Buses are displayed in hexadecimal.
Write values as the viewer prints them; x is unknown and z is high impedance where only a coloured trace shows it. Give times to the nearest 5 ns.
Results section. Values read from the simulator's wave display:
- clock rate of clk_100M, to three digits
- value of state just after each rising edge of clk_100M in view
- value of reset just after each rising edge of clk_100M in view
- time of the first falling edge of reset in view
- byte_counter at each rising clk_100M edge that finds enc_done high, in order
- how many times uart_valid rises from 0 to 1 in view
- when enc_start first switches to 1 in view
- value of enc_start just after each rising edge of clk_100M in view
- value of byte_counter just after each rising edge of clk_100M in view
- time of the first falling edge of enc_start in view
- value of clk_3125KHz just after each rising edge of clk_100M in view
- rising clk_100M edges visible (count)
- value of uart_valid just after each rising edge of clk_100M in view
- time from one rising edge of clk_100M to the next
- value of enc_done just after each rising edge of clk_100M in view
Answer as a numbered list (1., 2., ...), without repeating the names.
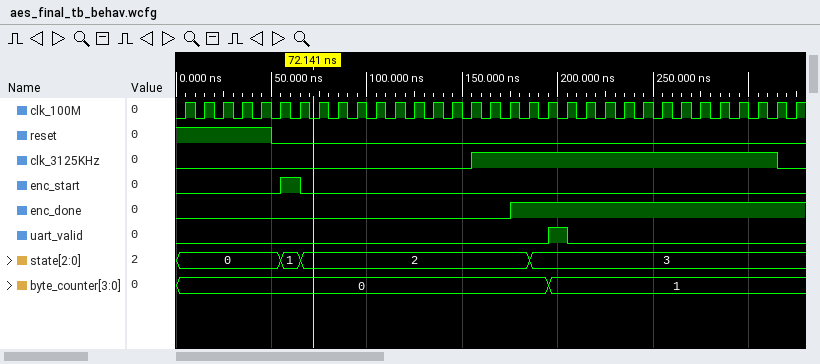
1. 100 MHz
2. 0, 0, 0, 0, 0, 1, 2, 2, 2, 2, 2, 2, 2, 2, 2, 2, 2, 2, 3, 3, 3, 3, 3, 3, 3, 3, 3, 3, 3, 3, 3, 3, 3
3. 1 1 1 1 1 0 0 0 0 0 0 0 0 0 0 0 0 0 0 0 0 0 0 0 0 0 0 0 0 0 0 0 0
4. 50 ns
5. 0, 0, 1, 1, 1, 1, 1, 1, 1, 1, 1, 1, 1, 1, 1
6. 1
7. 55 ns
8. 0 0 0 0 0 1 0 0 0 0 0 0 0 0 0 0 0 0 0 0 0 0 0 0 0 0 0 0 0 0 0 0 0
9. 0, 0, 0, 0, 0, 0, 0, 0, 0, 0, 0, 0, 0, 0, 0, 0, 0, 0, 0, 1, 1, 1, 1, 1, 1, 1, 1, 1, 1, 1, 1, 1, 1
10. 65 ns
11. 0 0 0 0 0 0 0 0 0 0 0 0 0 0 0 1 1 1 1 1 1 1 1 1 1 1 1 1 1 1 1 0 0
12. 33
13. 0 0 0 0 0 0 0 0 0 0 0 0 0 0 0 0 0 0 0 1 0 0 0 0 0 0 0 0 0 0 0 0 0
14. 10 ns
15. 0 0 0 0 0 0 0 0 0 0 0 0 0 0 0 0 0 1 1 1 1 1 1 1 1 1 1 1 1 1 1 1 1
